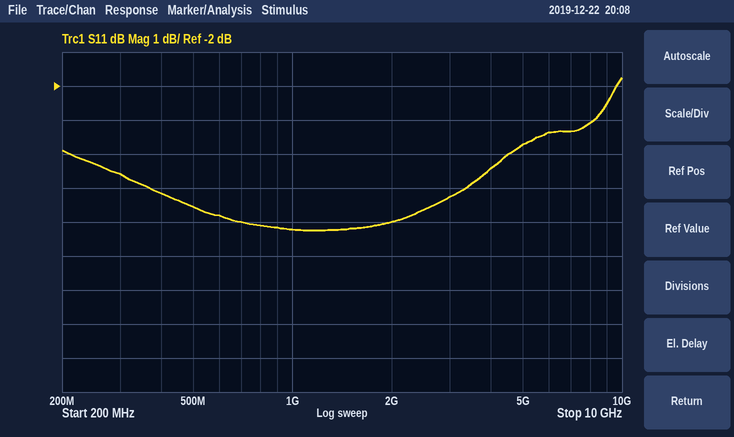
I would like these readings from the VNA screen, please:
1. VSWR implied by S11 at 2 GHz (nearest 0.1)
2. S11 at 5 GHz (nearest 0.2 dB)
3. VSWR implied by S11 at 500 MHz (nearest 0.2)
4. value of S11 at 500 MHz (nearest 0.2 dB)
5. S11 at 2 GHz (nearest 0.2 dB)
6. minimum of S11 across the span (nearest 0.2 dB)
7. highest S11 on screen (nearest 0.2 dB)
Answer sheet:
3.0
-3.8 dB
3.2
-5.6 dB
-6.0 dB
-6.2 dB
-1.8 dB
